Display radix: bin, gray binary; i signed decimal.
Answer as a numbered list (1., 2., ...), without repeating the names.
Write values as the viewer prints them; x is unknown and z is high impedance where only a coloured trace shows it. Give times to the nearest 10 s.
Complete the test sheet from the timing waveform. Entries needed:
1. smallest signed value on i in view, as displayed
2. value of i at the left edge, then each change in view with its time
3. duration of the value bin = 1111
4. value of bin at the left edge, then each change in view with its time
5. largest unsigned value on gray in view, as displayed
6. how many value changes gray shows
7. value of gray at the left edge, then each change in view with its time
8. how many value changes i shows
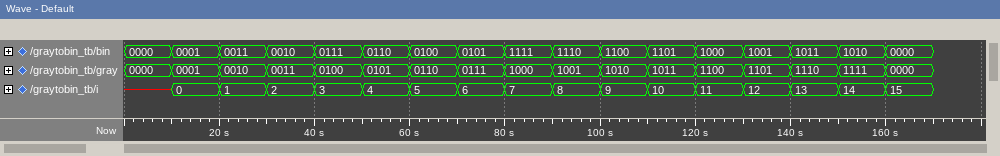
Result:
1. 0
2. x, 0 at 10 s, 1 at 20 s, 2 at 30 s, 3 at 40 s, 4 at 50 s, 5 at 60 s, 6 at 70 s, 7 at 80 s, 8 at 90 s, 9 at 100 s, 10 at 110 s, 11 at 120 s, 12 at 130 s, 13 at 140 s, 14 at 150 s, 15 at 160 s
3. 10 s
4. 0000, 0001 at 10 s, 0011 at 20 s, 0010 at 30 s, 0111 at 40 s, 0110 at 50 s, 0100 at 60 s, 0101 at 70 s, 1111 at 80 s, 1110 at 90 s, 1100 at 100 s, 1101 at 110 s, 1000 at 120 s, 1001 at 130 s, 1011 at 140 s, 1010 at 150 s, 0000 at 160 s
5. 1111
6. 16
7. 0000, 0001 at 10 s, 0010 at 20 s, 0011 at 30 s, 0100 at 40 s, 0101 at 50 s, 0110 at 60 s, 0111 at 70 s, 1000 at 80 s, 1001 at 90 s, 1010 at 100 s, 1011 at 110 s, 1100 at 120 s, 1101 at 130 s, 1110 at 140 s, 1111 at 150 s, 0000 at 160 s
8. 16
